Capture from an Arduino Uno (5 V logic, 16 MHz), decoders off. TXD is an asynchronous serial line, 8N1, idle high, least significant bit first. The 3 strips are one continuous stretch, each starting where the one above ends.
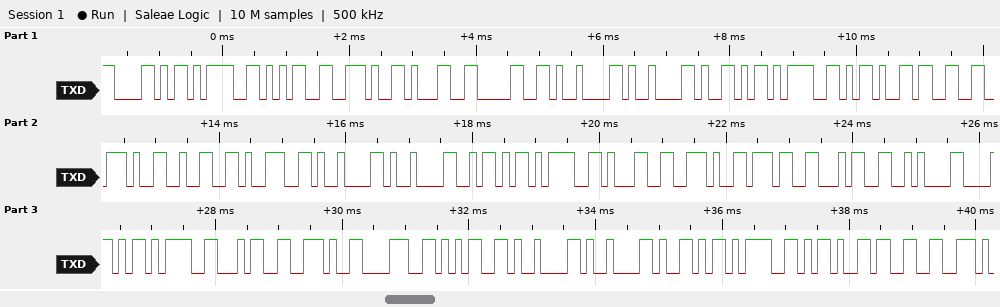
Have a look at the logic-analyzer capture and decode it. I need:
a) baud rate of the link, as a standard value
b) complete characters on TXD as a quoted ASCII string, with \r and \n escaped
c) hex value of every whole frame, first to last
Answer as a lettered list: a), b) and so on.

a) 9600 baud
b) "X=5.10\t\tY=-3.29\t\tZ=1.74\nX=4.85\t\tY=-3"
c) 0x58 0x3D 0x35 0x2E 0x31 0x30 0x09 0x09 0x59 0x3D 0x2D 0x33 0x2E 0x32 0x39 0x09 0x09 0x5A 0x3D 0x31 0x2E 0x37 0x34 0x0A 0x58 0x3D 0x34 0x2E 0x38 0x35 0x09 0x09 0x59 0x3D 0x2D 0x33
